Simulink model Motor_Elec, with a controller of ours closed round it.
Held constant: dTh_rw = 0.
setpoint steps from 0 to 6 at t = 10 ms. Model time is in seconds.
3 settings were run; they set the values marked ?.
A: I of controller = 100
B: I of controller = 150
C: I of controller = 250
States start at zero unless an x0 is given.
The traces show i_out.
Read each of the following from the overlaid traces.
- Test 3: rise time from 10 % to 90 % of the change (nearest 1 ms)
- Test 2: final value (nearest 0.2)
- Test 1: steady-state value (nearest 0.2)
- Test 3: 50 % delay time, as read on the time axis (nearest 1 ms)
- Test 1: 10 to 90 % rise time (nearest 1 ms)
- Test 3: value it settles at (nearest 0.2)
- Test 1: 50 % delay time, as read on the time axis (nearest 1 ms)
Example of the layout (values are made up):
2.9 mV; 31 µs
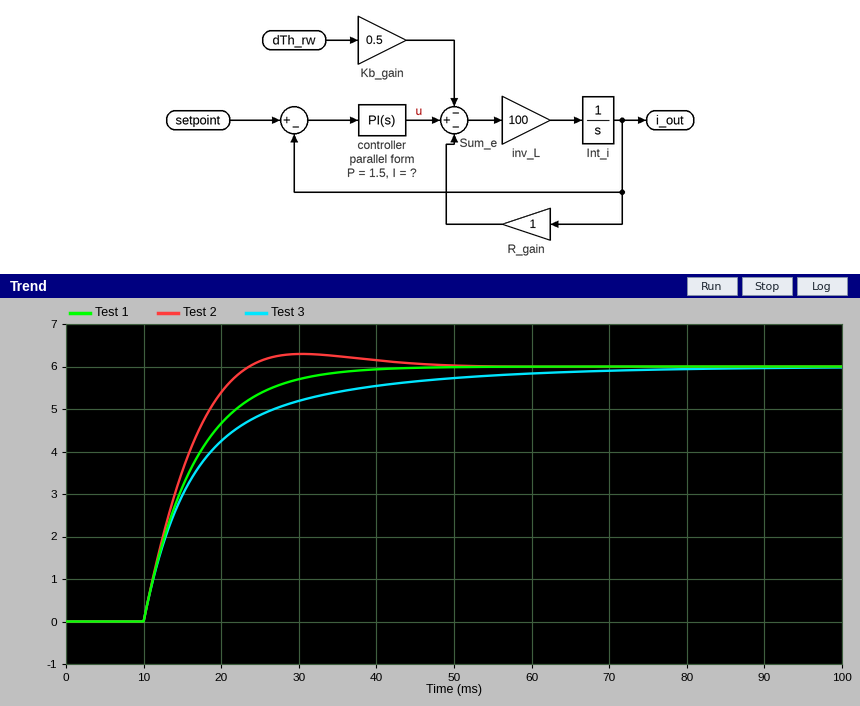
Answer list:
24 ms; 6.0; 6.0; 15 ms; 15 ms; 6.0; 15 ms
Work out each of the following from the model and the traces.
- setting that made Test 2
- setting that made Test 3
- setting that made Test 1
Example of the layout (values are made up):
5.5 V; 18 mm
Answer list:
C; A; B
